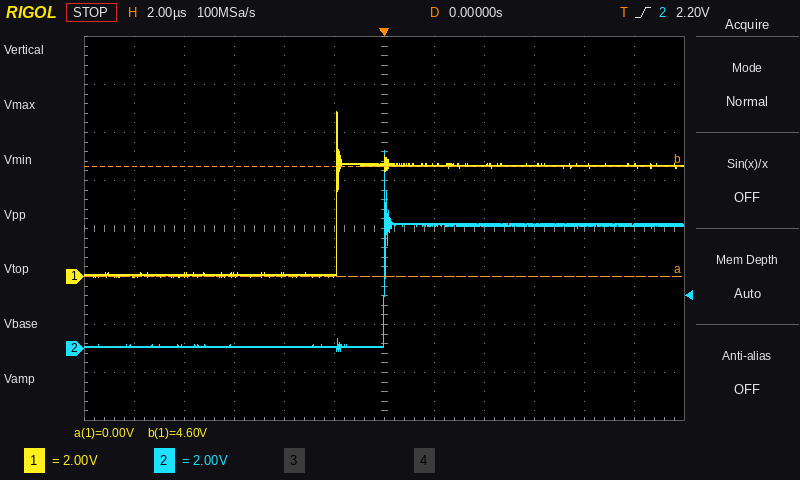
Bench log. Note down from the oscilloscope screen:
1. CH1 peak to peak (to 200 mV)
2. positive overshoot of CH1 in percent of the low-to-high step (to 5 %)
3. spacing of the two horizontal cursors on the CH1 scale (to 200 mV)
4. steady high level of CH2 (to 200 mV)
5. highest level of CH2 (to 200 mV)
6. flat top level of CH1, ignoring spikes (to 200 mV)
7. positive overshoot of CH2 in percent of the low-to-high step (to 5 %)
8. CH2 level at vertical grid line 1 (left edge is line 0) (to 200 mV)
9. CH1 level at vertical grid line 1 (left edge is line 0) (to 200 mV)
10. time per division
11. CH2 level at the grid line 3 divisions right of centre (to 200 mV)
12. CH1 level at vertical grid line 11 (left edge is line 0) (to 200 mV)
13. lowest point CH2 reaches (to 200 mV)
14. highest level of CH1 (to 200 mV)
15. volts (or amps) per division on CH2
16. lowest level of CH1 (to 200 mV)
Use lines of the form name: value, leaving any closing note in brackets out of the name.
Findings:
CH1 peak to peak: 6.8 V
positive overshoot of CH1 in percent of the low-to-high step: 50 %
spacing of the two horizontal cursors on the CH1 scale: 4.6 V
steady high level of CH2: 5.2 V
highest level of CH2: 8.2 V
flat top level of CH1, ignoring spikes: 4.6 V
positive overshoot of CH2 in percent of the low-to-high step: 60 %
CH2 level at vertical grid line 1 (left edge is line 0): 0.0 V
CH1 level at vertical grid line 1 (left edge is line 0): 0.0 V
time per division: 2 µs
CH2 level at the grid line 3 divisions right of centre: 5.2 V
CH1 level at vertical grid line 11 (left edge is line 0): 4.6 V
lowest point CH2 reaches: 0.0 V
highest level of CH1: 6.8 V
volts (or amps) per division on CH2: 2 V
lowest level of CH1: 0.0 V
